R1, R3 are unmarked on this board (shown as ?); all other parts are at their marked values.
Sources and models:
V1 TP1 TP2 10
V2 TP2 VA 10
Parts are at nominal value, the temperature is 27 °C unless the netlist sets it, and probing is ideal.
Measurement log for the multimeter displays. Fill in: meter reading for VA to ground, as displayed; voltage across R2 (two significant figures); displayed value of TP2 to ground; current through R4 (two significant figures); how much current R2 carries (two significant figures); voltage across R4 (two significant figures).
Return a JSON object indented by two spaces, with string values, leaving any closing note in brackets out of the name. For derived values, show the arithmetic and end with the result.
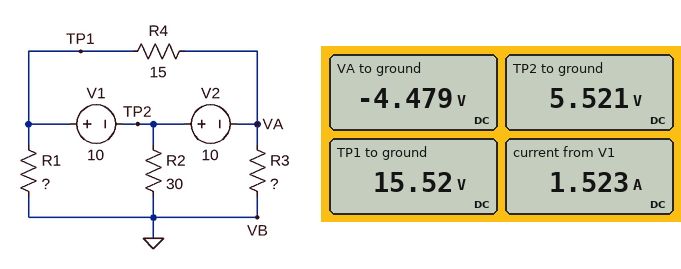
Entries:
{
  "meter reading for VA to ground, as displayed": "-4.479 V",
  "voltage across R2": "5.521 V = 5.5 V",
  "displayed value of TP2 to ground": "5.521 V",
  "current through R4": "(15.52 V - (-4.479 V)) / 15 Ω = 1.3 A",
  "how much current R2 carries": "(5.521 V) / 30 Ω = 180 mA",
  "voltage across R4": "15.52 V - (-4.479 V) = 20 V"
}
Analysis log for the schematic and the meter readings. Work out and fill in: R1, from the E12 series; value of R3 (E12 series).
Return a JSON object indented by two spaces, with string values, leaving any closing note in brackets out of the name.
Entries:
{
  "R1, from the E12 series": "82 Ω",
  "value of R3": "12 Ω"
}
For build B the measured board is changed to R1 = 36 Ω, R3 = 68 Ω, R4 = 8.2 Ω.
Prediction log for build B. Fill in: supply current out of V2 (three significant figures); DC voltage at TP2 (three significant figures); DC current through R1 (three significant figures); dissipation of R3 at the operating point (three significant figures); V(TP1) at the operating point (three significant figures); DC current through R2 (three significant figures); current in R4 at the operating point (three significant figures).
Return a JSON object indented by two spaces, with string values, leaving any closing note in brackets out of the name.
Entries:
{
  "supply current out of V2": "2.61 A",
  "DC voltage at TP2": "-1.72 V",
  "DC current through R1": "230 mA",
  "dissipation of R3 at the operating point": "2.02 W",
  "V(TP1) at the operating point": "8.28 V",
  "DC current through R2": "57.5 mA",
  "current in R4 at the operating point": "2.44 A"
}
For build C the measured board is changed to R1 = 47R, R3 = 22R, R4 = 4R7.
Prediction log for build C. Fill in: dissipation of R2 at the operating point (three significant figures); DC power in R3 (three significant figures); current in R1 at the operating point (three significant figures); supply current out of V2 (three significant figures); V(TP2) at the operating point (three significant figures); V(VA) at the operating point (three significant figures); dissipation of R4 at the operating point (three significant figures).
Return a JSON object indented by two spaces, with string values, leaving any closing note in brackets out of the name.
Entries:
{
  "dissipation of R2 at the operating point": "195 mW",
  "DC power in R3": "2.61 W",
  "current in R1 at the operating point": "264 mA",
  "supply current out of V2": "4.60 A",
  "V(TP2) at the operating point": "2.42 V",
  "V(VA) at the operating point": "-7.58 V",
  "dissipation of R4 at the operating point": "85.1 W"
}
